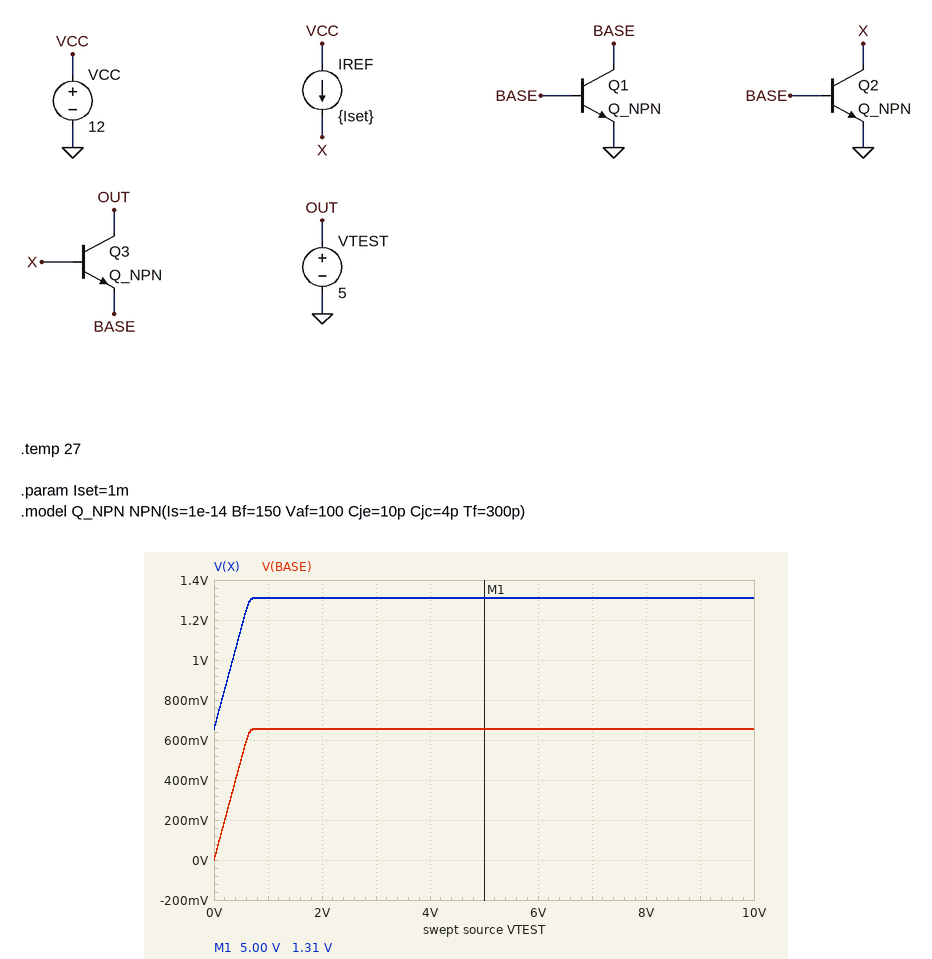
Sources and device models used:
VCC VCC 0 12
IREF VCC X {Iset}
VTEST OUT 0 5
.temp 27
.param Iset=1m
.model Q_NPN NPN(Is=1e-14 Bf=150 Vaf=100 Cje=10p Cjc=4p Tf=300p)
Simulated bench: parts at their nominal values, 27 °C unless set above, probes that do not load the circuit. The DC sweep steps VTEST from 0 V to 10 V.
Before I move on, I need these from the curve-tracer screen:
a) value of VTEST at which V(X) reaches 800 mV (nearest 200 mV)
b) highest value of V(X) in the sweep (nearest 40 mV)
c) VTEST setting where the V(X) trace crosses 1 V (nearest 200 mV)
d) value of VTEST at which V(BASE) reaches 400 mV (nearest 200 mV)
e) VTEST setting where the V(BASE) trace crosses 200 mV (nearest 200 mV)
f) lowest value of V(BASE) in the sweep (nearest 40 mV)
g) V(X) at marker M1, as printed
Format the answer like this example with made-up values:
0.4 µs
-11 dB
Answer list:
200 mV
1.32 V
400 mV
400 mV
200 mV
0 V
1.31 V
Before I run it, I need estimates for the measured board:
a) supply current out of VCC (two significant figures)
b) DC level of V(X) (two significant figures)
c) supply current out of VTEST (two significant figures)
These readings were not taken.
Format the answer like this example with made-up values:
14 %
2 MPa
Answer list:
1.0 mA
1.3 V
990 µA
